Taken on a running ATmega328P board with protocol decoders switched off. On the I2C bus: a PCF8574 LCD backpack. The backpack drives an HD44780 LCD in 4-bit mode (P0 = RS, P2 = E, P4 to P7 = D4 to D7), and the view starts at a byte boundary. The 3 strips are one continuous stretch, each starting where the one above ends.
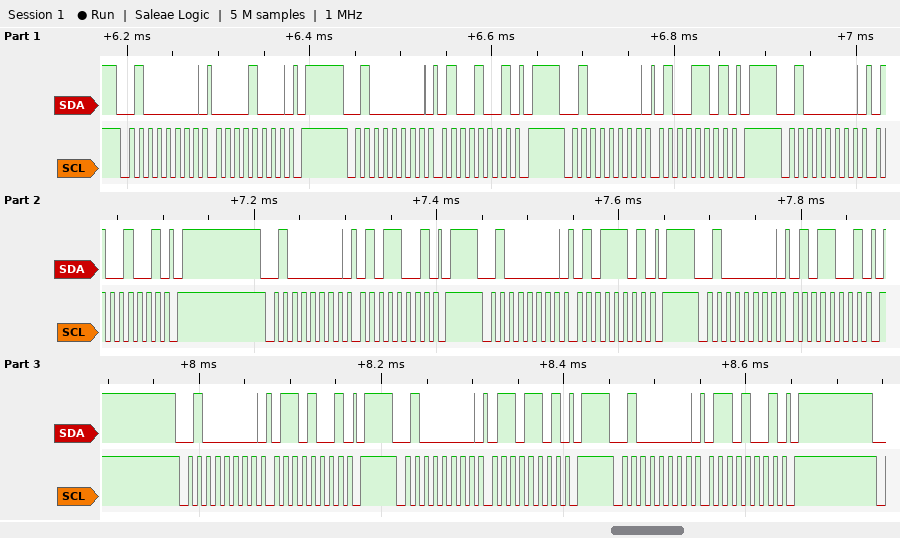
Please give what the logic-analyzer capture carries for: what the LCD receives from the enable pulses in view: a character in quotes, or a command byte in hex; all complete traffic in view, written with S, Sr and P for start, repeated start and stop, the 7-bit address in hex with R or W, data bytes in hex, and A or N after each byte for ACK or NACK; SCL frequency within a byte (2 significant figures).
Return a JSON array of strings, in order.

["'E'", "S 20W A 08 A P S 20W A 49 A P S 20W A 4D A P S 20W A 49 A P S 20W A 59 A P S 20W A 5D A P S 20W A 59 A P S 20W A 69 A P S 20W A 6D A P S 20W A 69 A P", "100 kHz"]
